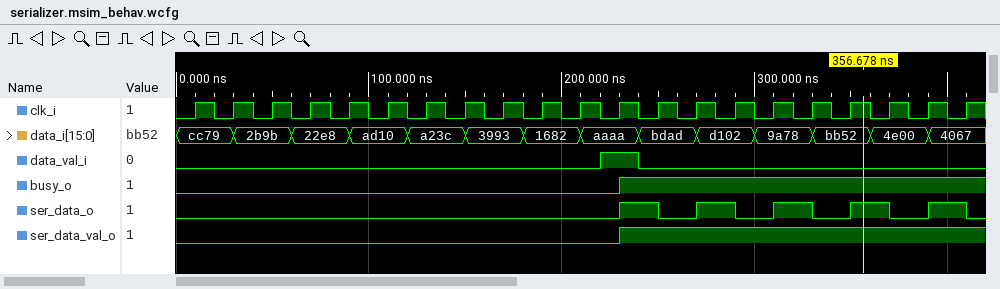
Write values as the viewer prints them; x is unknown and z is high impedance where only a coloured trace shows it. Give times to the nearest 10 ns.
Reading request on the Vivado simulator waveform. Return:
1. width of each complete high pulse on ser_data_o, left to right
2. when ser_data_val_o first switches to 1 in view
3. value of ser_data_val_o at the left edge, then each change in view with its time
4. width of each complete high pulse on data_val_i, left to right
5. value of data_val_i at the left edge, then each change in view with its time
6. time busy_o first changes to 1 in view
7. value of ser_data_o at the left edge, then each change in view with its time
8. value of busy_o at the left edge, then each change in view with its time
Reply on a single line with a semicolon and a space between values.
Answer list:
20 ns, 20 ns, 20 ns, 20 ns, 20 ns; 230 ns; 0, 1 at 230 ns; 20 ns; 0, 1 at 220 ns, 0 at 240 ns; 230 ns; 0, 1 at 230 ns, 0 at 250 ns, 1 at 270 ns, 0 at 290 ns, 1 at 310 ns, 0 at 330 ns, 1 at 350 ns, 0 at 370 ns, 1 at 390 ns, 0 at 410 ns; 0, 1 at 230 ns
